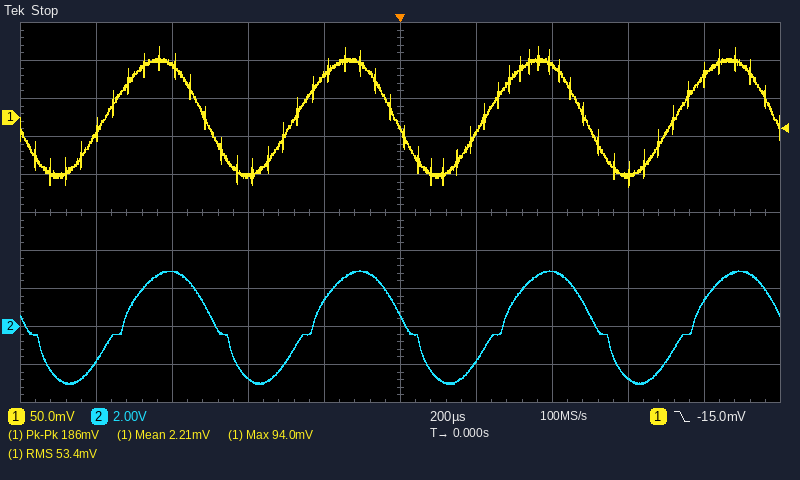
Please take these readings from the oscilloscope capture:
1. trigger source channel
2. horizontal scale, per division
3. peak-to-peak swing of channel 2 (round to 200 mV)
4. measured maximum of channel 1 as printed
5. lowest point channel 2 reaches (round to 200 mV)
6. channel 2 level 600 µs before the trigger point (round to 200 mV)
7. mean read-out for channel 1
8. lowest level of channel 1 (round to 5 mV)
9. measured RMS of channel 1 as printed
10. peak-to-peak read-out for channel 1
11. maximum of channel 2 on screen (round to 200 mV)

channel 1
200 µs
6.0 V
94.0 mV
-3.0 V
2.8 V
2.21 mV
-90 mV
53.4 mV
186 mV
3.0 V
